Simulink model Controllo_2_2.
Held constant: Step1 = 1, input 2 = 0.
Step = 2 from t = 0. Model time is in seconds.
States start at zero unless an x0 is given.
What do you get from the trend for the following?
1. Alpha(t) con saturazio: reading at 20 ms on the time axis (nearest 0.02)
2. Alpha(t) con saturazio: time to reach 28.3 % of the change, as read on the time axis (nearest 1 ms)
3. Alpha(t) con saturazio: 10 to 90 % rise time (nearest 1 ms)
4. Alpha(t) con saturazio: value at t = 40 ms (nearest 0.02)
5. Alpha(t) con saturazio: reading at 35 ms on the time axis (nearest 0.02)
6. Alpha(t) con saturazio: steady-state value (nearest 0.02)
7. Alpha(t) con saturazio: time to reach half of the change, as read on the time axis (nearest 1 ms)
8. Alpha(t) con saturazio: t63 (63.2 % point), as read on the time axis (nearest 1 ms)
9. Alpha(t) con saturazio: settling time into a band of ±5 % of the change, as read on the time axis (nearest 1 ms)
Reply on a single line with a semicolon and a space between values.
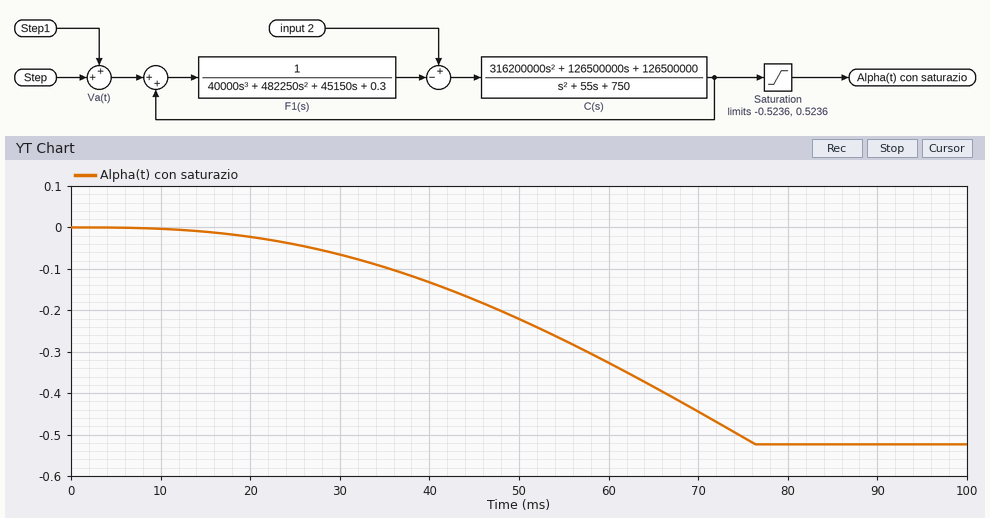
-0.02; 42 ms; 45 ms; -0.14; -0.10; -0.52; 54 ms; 60 ms; 74 ms
